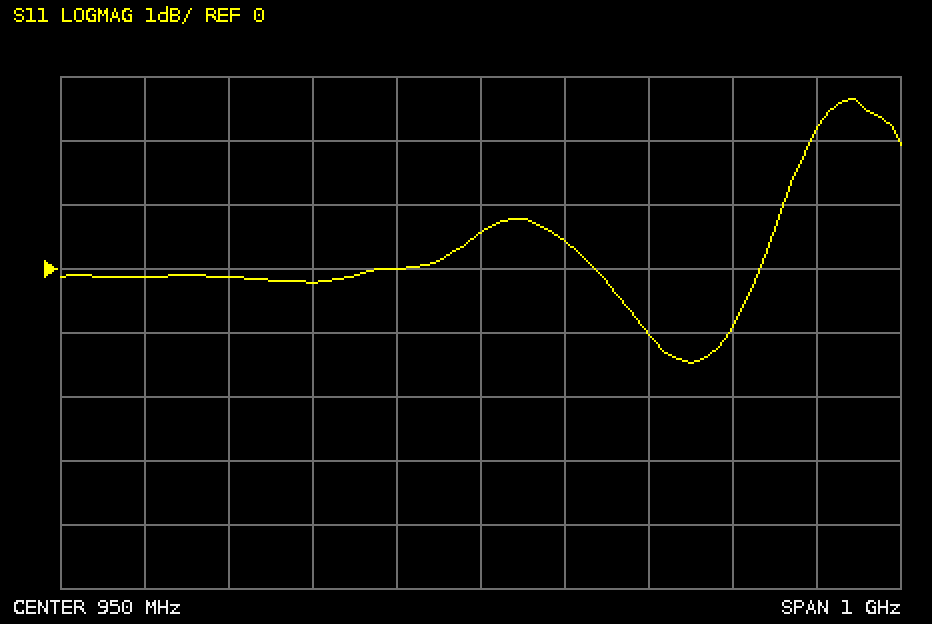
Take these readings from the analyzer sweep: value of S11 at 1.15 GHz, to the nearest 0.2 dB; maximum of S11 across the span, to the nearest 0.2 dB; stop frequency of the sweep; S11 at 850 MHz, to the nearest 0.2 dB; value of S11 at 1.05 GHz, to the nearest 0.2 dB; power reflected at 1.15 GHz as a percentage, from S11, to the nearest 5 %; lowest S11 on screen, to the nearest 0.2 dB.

-1.0 dB
2.6 dB
1.45 GHz
0.0 dB
0.4 dB
80 %
-1.4 dB
